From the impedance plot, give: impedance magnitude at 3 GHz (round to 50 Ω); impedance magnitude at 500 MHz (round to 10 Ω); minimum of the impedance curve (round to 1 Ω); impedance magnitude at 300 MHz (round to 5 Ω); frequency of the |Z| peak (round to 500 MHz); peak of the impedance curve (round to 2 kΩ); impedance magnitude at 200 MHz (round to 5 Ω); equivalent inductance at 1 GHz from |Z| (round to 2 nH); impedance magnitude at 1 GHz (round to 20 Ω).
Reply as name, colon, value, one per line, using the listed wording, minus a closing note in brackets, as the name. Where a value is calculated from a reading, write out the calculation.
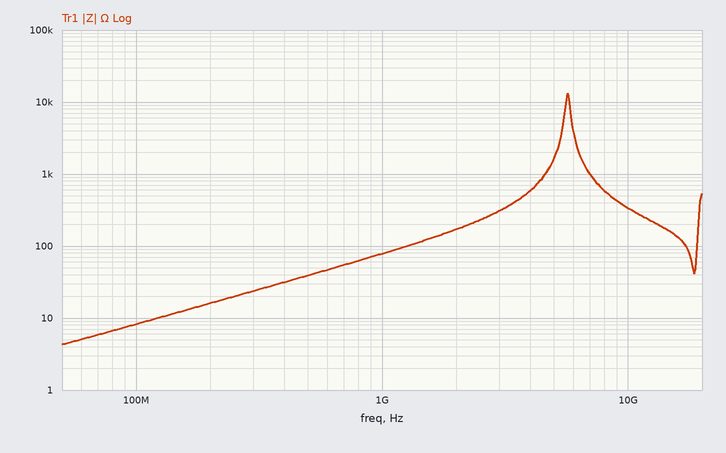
impedance magnitude at 3 GHz: 300 Ω
impedance magnitude at 500 MHz: 40 Ω
minimum of the impedance curve: 4 Ω
impedance magnitude at 300 MHz: 25 Ω
frequency of the |Z| peak: 5.5 GHz
peak of the impedance curve: 14 kΩ
impedance magnitude at 200 MHz: 15 Ω
equivalent inductance at 1 GHz from |Z|: L = 80 Ω/(2π × 1 GHz) ≈ 12.7 nH, so 12 nH to the nearest 2 nH
impedance magnitude at 1 GHz: 80 Ω
